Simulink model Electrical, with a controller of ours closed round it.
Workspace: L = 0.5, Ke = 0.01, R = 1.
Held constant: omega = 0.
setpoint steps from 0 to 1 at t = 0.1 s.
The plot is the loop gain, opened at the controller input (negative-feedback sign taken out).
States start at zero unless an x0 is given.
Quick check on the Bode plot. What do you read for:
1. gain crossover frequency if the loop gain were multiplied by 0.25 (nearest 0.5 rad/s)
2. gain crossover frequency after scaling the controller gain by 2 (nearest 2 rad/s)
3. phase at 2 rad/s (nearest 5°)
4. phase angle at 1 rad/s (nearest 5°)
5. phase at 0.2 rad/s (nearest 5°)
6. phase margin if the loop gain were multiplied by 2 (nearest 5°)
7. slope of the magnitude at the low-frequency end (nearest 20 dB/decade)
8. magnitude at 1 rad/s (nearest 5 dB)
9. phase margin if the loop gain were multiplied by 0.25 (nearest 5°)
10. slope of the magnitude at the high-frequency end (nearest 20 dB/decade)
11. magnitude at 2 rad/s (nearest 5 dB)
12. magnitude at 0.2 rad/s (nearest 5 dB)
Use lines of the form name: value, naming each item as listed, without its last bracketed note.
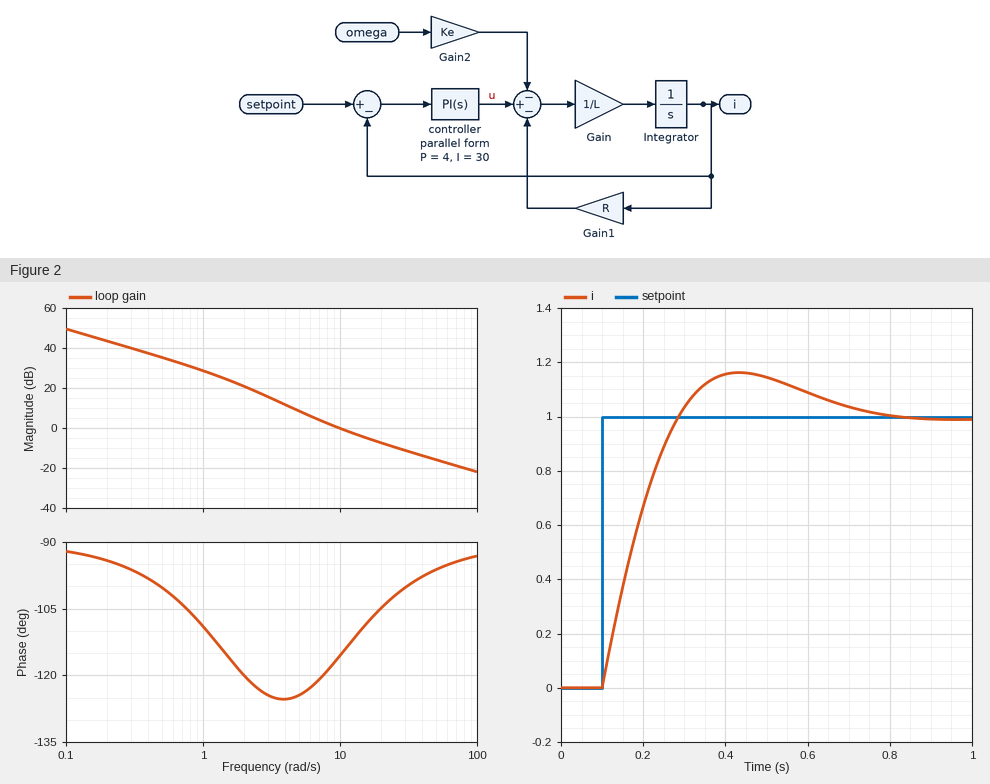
gain crossover frequency if the loop gain were multiplied by 0.25: 4.0 rad/s
gain crossover frequency after scaling the controller gain by 2: 18 rad/s
phase at 2 rad/s: -120°
phase angle at 1 rad/s: -110°
phase at 0.2 rad/s: -95°
phase margin if the loop gain were multiplied by 2: 75°
slope of the magnitude at the low-frequency end: -20 dB/decade
magnitude at 1 rad/s: 30 dB
phase margin if the loop gain were multiplied by 0.25: 55°
slope of the magnitude at the high-frequency end: -20 dB/decade
magnitude at 2 rad/s: 20 dB
magnitude at 0.2 rad/s: 45 dB
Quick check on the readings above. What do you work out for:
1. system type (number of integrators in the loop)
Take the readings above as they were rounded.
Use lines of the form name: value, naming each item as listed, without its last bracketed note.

system type: 1
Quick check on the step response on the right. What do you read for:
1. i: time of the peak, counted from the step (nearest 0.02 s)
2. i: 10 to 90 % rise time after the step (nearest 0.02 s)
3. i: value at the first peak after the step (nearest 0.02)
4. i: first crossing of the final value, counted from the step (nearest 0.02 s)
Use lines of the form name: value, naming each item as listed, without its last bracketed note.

i: time of the peak, counted from the step: 0.34 s
i: 10 to 90 % rise time after the step: 0.14 s
i: value at the first peak after the step: 1.16
i: first crossing of the final value, counted from the step: 0.18 s
